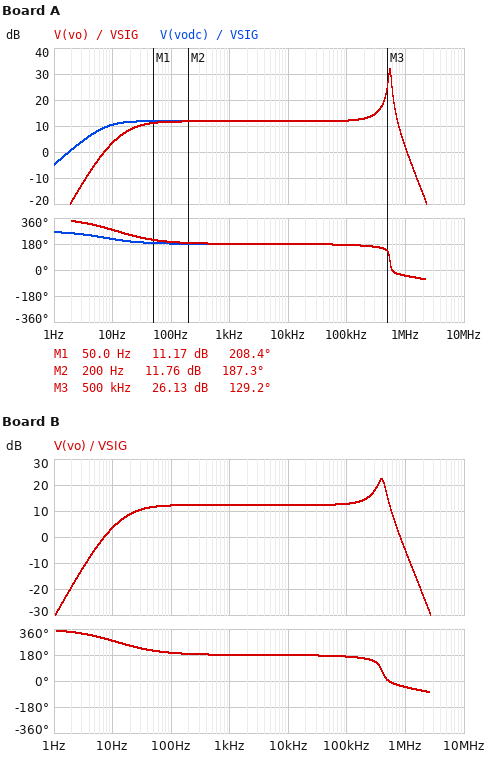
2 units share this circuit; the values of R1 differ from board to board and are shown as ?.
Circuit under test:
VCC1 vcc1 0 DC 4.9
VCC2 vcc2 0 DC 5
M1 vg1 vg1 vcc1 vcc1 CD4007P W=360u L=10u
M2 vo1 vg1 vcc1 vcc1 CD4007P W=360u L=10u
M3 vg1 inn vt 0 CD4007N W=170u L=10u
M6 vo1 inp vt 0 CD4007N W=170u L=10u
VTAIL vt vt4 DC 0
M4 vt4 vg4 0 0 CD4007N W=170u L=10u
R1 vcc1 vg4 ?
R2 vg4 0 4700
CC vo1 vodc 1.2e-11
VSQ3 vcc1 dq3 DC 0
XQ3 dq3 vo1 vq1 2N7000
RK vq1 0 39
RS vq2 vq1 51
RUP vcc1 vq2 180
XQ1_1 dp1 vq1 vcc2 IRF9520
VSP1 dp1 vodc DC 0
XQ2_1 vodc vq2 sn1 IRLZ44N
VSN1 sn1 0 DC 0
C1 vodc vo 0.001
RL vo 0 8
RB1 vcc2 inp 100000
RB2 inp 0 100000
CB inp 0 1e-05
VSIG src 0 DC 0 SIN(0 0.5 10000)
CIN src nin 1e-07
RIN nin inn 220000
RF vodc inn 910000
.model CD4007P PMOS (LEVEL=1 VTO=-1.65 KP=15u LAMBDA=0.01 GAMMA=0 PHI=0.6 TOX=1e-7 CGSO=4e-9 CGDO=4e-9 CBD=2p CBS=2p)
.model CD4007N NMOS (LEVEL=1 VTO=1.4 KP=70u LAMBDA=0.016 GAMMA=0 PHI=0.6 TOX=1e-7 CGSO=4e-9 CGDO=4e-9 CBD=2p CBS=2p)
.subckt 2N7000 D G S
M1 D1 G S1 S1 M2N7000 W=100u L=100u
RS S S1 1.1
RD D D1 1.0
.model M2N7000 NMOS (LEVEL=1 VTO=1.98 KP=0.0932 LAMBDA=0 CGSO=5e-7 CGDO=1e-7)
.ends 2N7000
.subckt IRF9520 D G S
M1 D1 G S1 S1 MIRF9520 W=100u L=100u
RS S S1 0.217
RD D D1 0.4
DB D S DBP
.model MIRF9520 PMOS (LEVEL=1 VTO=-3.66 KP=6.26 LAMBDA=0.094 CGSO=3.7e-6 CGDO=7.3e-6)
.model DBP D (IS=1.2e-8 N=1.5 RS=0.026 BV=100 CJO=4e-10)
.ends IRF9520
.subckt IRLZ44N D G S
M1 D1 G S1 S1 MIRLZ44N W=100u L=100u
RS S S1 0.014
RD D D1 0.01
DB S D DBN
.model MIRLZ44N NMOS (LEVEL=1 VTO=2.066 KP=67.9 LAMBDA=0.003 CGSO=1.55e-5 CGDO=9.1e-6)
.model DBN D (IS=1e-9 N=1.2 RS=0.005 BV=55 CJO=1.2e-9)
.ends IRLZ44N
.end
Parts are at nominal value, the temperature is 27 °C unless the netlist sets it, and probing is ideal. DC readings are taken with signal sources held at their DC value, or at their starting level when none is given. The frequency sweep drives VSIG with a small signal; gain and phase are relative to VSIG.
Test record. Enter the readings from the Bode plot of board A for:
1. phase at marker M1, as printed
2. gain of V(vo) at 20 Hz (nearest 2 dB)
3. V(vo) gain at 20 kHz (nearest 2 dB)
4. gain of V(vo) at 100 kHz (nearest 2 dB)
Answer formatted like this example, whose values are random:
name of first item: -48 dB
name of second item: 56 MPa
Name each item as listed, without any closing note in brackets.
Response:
phase at marker M1, as printed: 208.4 deg
gain of V(vo) at 20 Hz: 8 dB
V(vo) gain at 20 kHz: 12 dB
gain of V(vo) at 100 kHz: 12 dB
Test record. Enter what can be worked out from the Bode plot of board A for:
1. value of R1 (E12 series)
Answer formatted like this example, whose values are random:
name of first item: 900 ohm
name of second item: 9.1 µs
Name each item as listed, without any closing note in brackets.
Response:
value of R1: 2.7 kΩ
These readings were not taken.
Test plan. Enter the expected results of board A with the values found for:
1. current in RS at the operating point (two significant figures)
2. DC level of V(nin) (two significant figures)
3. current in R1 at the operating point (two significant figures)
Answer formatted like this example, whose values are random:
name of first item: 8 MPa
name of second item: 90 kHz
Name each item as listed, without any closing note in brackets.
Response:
current in RS at the operating point: 16 mA
DC level of V(nin): 2.5 V
current in R1 at the operating point: 660 µA
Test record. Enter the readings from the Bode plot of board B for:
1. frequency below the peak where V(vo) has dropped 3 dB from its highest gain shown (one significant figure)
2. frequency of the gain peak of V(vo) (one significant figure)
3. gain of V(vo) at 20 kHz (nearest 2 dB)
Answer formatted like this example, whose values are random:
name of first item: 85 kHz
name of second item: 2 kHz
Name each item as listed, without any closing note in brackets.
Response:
frequency below the peak where V(vo) has dropped 3 dB from its highest gain shown: 300 kHz
frequency of the gain peak of V(vo): 400 kHz
gain of V(vo) at 20 kHz: 12 dB
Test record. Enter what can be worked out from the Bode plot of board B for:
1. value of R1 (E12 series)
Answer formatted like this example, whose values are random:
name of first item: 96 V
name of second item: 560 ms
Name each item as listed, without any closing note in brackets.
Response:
value of R1: 8.2 kΩ
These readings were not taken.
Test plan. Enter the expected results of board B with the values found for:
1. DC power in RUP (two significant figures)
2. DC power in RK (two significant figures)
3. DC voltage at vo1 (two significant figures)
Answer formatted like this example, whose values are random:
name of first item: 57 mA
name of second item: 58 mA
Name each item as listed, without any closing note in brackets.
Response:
DC power in RUP: 44 mW
DC power in RK: 42 mW
DC voltage at vo1: 3.9 V
